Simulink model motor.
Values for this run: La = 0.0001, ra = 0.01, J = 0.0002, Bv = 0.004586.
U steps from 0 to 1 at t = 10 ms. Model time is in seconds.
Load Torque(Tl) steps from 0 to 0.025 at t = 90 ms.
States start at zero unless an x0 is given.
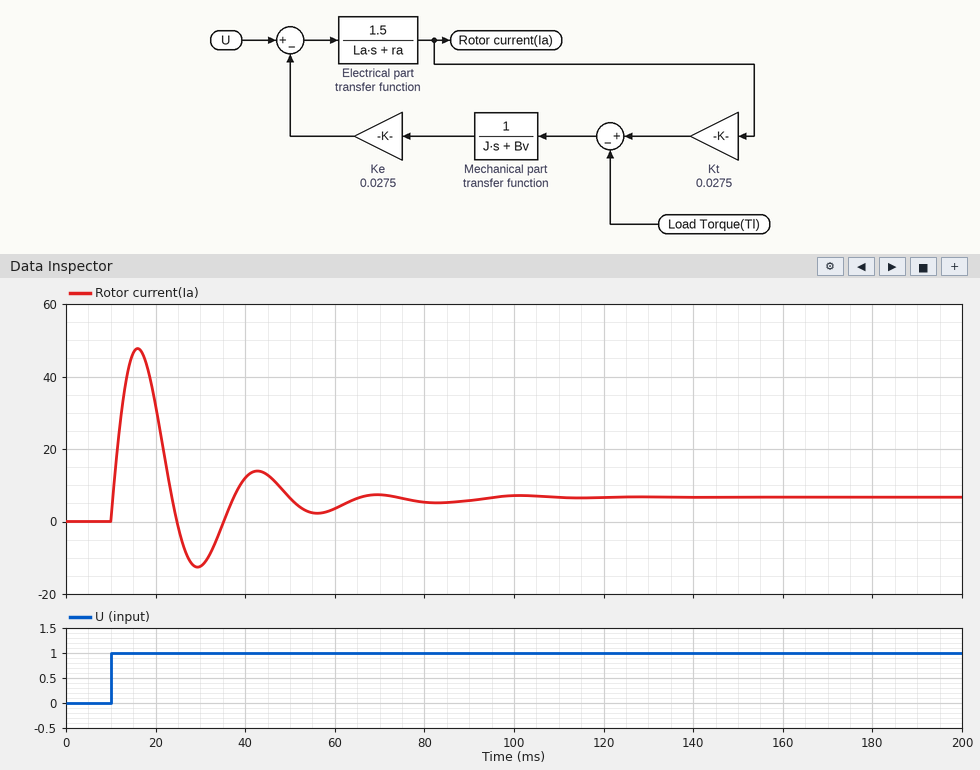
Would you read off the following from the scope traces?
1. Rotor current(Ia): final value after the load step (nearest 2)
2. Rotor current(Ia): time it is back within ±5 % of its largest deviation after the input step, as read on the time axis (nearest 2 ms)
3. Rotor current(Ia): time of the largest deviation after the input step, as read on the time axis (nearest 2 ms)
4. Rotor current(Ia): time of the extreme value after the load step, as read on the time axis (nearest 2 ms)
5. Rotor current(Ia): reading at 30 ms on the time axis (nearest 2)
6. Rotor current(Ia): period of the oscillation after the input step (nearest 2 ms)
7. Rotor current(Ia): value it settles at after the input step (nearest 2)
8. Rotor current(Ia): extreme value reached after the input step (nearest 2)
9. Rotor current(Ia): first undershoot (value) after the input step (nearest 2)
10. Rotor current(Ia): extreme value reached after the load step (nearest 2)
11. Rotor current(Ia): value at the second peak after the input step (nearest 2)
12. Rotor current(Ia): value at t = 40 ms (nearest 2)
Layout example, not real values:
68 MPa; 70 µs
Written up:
6; 60 ms; 16 ms; 102 ms; -12; 26 ms; 6; 48; -12; 8; 14; 12
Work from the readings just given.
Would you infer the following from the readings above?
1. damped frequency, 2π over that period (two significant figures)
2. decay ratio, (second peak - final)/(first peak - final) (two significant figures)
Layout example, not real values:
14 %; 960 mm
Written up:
0.24 rad/ms; 0.19
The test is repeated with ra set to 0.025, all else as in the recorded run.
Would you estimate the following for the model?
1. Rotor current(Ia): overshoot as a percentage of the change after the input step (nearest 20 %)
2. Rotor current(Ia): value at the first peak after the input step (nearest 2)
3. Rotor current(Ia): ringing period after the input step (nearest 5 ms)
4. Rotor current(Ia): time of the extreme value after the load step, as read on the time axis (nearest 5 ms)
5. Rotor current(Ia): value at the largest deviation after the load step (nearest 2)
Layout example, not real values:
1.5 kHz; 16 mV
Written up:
520 %; 34; 30 ms; 105 ms; 6
